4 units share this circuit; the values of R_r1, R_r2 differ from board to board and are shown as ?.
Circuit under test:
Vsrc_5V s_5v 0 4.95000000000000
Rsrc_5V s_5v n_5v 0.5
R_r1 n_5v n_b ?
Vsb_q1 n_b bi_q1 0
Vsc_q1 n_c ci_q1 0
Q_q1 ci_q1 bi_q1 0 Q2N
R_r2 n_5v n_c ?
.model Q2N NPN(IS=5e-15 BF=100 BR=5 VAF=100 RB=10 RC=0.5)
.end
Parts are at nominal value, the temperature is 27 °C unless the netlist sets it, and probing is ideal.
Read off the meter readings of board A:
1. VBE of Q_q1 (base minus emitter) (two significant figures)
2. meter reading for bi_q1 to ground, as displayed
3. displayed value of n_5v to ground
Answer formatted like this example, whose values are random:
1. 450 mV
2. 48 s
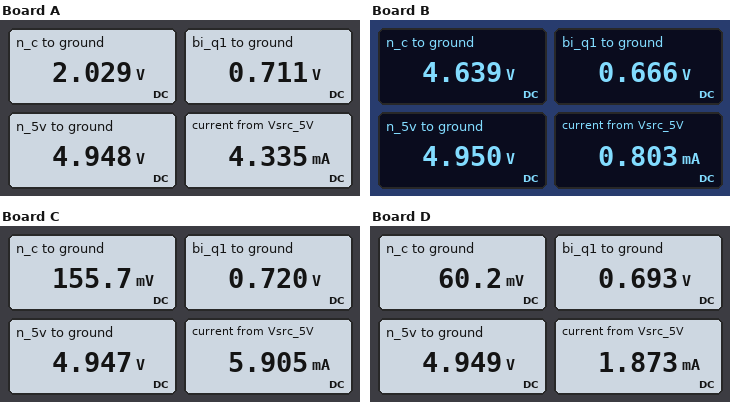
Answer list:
1. 710 mV
2. 0.711 V
3. 4.948 V
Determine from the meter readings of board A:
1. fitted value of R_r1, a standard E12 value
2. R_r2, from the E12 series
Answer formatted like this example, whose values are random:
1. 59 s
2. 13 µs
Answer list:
1. 100 kΩ
2. 680 Ω
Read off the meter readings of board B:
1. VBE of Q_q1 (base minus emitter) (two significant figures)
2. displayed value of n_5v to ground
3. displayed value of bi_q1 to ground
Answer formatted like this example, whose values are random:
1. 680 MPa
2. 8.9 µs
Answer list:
1. 670 mV
2. 4.950 V
3. 0.666 V
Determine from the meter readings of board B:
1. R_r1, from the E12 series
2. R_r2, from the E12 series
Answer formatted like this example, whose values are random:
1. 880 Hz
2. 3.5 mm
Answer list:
1. 560 kΩ
2. 390 Ω
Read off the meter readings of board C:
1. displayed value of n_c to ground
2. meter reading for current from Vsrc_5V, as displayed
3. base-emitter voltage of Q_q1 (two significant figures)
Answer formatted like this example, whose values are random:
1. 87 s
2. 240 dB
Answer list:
1. 155.7 mV
2. 5.905 mA
3. 720 mV
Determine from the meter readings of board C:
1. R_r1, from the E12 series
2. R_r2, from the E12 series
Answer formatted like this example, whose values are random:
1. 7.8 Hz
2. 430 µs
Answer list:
1. 68 kΩ
2. 820 Ω
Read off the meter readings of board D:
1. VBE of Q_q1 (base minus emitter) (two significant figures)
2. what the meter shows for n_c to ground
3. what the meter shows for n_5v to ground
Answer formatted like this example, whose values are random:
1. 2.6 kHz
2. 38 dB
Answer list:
1. 690 mV
2. 60.2 mV
3. 4.949 V
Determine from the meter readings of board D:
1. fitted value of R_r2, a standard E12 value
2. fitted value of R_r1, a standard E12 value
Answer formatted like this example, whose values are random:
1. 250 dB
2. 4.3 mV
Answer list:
1. 2.7 kΩ
2. 68 kΩ
